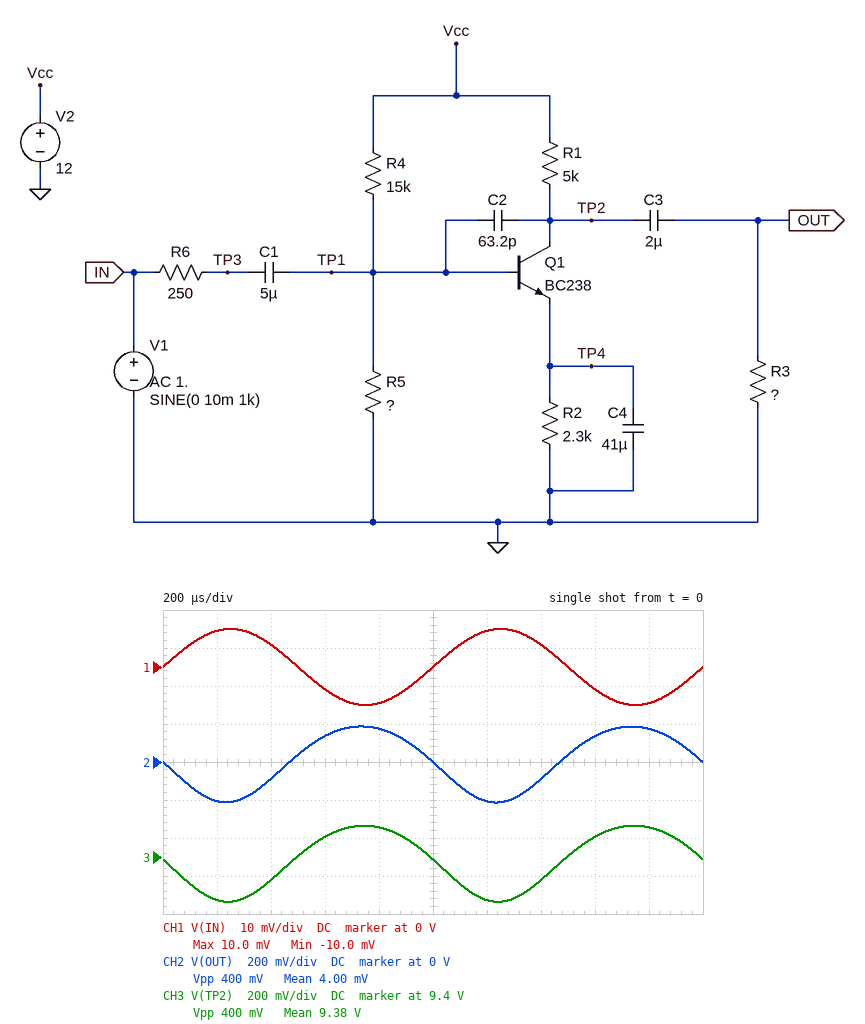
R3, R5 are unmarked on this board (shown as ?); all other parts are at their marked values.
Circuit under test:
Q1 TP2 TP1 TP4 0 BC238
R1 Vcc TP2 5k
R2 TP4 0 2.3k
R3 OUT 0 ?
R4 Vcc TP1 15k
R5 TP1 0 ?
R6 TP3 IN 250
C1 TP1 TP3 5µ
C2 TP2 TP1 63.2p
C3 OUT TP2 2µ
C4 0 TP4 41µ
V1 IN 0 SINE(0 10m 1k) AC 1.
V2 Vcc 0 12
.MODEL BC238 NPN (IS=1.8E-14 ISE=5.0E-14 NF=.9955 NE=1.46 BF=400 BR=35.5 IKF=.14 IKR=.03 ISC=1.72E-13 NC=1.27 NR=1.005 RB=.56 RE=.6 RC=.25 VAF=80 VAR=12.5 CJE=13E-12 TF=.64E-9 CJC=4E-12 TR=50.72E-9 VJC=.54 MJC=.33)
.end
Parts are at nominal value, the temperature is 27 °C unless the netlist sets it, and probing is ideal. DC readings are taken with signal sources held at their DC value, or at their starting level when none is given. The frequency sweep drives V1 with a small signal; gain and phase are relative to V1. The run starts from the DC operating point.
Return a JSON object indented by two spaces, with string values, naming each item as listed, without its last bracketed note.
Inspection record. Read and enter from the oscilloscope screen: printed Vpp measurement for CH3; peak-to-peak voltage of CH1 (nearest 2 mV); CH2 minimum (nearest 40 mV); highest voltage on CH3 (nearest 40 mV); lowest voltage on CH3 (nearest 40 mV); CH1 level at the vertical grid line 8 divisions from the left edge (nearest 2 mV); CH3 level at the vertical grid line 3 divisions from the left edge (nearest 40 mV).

{
  "printed Vpp measurement for CH3": "400 mV",
  "peak-to-peak voltage of CH1": "20 mV",
  "CH2 minimum": "-200 mV",
  "highest voltage on CH3": "9.56 V",
  "lowest voltage on CH3": "9.16 V",
  "CH1 level at the vertical grid line 8 divisions from the left edge": "-6 mV",
  "CH3 level at the vertical grid line 3 divisions from the left edge": "9.52 V"
}
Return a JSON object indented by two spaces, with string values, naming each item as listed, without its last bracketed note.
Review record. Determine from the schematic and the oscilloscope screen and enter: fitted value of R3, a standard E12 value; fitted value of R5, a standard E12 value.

{
  "fitted value of R3, a standard E12 value": "1.5 kΩ",
  "fitted value of R5, a standard E12 value": "2.7 kΩ"
}
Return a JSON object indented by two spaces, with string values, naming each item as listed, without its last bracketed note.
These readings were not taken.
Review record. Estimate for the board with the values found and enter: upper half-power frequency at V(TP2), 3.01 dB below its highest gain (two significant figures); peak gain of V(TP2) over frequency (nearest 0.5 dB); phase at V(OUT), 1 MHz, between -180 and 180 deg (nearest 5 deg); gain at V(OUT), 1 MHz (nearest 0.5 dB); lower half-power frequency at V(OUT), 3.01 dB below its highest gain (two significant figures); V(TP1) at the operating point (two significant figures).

{
  "upper half-power frequency at V(TP2), 3.01 dB below its highest gain": "380 kHz",
  "peak gain of V(TP2) over frequency": "26.0 dB",
  "phase at V(OUT), 1 MHz, between -180 and 180 deg": "110 deg",
  "gain at V(OUT), 1 MHz": "17.0 dB",
  "lower half-power frequency at V(OUT), 3.01 dB below its highest gain": "83 Hz",
  "V(TP1) at the operating point": "1.8 V"
}
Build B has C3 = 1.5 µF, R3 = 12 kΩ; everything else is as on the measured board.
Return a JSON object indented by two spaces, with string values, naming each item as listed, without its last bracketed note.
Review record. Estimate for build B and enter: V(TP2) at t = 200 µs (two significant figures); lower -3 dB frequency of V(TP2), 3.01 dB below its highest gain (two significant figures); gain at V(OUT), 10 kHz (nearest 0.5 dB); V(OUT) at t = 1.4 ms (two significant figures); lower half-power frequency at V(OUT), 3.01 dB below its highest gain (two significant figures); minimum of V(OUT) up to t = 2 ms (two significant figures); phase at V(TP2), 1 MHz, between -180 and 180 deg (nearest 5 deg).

{
  "V(TP2) at t = 200 µs": "8.8 V",
  "lower -3 dB frequency of V(TP2), 3.01 dB below its highest gain": "80 Hz",
  "gain at V(OUT), 10 kHz": "35.5 dB",
  "V(OUT) at t = 1.4 ms": "-280 mV",
  "lower half-power frequency at V(OUT), 3.01 dB below its highest gain": "81 Hz",
  "minimum of V(OUT) up to t = 2 ms": "-640 mV",
  "phase at V(TP2), 1 MHz, between -180 and 180 deg": "95 deg"
}
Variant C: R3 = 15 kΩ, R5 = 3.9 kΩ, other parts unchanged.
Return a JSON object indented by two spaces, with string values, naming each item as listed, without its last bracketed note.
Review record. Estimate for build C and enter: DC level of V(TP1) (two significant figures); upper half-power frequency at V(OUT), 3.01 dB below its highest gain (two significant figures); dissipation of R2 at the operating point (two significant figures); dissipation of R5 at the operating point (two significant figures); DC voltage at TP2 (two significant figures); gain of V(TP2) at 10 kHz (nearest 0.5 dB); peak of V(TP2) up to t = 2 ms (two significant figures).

{
  "DC level of V(TP1)": "2.5 V",
  "upper half-power frequency at V(OUT), 3.01 dB below its highest gain": "86 kHz",
  "dissipation of R2 at the operating point": "1.5 mW",
  "dissipation of R5 at the operating point": "1.6 mW",
  "DC voltage at TP2": "8.0 V",
  "gain of V(TP2) at 10 kHz": "40.0 dB",
  "peak of V(TP2) up to t = 2 ms": "8.9 V"
}
